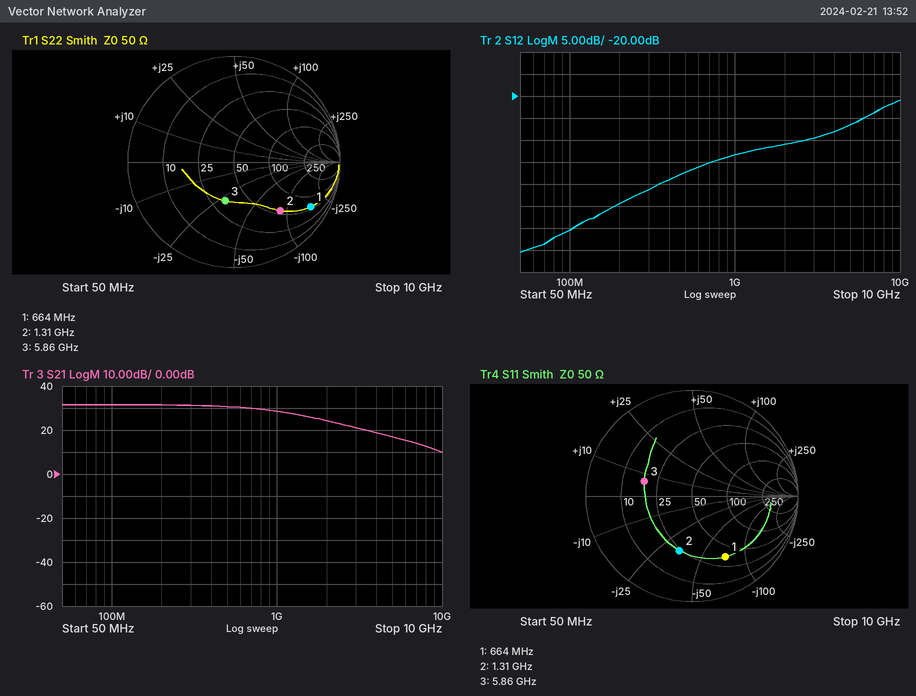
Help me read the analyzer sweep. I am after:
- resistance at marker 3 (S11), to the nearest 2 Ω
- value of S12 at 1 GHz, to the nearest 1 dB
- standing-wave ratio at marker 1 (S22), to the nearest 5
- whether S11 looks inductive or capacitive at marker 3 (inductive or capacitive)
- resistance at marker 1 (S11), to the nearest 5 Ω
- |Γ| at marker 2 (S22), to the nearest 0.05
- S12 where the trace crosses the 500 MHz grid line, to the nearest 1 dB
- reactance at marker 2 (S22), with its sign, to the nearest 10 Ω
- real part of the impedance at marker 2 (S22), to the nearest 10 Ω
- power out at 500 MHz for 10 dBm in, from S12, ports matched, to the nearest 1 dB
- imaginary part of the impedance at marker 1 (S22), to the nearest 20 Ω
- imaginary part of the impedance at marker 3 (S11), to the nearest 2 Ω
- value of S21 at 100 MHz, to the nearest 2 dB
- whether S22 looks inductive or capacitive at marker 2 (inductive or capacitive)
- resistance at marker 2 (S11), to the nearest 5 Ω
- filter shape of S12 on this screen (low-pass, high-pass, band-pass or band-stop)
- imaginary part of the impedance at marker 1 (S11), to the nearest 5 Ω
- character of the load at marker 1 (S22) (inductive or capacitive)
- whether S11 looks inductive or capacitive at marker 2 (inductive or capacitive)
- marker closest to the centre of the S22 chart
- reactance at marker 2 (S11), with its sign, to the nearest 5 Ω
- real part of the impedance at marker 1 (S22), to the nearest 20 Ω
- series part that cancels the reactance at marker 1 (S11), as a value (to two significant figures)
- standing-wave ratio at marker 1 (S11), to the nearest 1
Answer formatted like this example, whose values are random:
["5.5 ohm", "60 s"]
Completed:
["18 Ω", "-33 dB", "10", "inductive", "35 Ω", "0.65", "-37 dB", "-90 Ω", "60 Ω", "-27 dBm", "-160 Ω", "+6 Ω", "32 dB", "capacitive", "25 Ω", "high-pass", "-70 Ω", "capacitive", "capacitive", "marker 3", "-35 Ω", "60 Ω", "17 nH", "5"]
